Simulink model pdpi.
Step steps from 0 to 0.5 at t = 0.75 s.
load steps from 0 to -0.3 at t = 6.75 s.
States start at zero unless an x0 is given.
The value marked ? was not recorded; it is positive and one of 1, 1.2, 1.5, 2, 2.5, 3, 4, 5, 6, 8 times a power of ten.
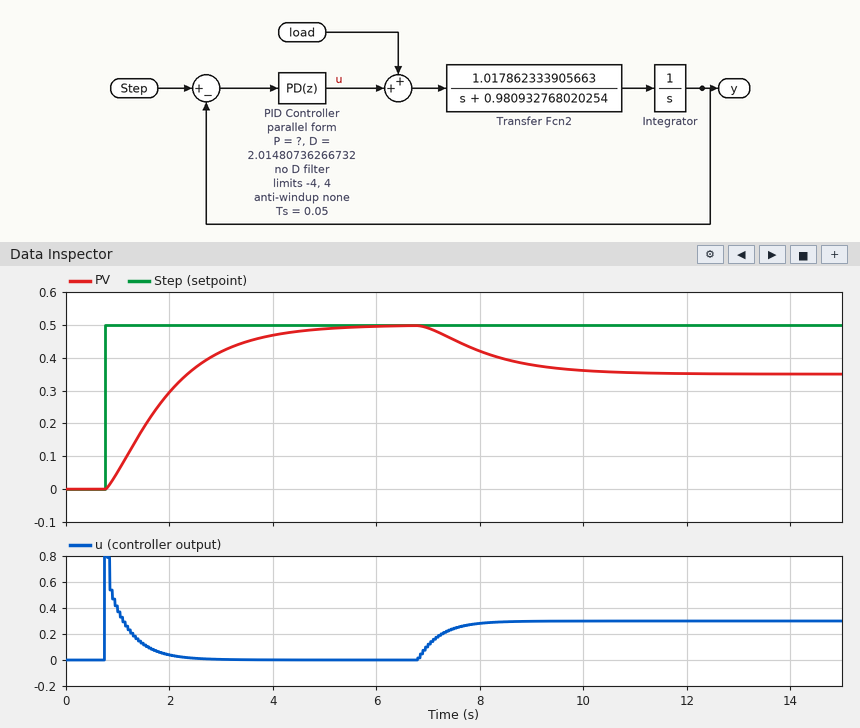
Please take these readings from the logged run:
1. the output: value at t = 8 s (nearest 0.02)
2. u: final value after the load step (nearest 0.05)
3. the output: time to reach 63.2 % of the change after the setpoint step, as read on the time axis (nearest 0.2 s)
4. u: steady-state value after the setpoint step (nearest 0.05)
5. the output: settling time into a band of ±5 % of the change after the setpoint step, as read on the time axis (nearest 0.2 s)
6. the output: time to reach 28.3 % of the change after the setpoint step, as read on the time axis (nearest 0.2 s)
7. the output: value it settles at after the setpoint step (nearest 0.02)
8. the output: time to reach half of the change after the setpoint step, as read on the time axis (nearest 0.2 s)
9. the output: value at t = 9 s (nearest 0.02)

0.42
0.30
2.2 s
0.00
4.2 s
1.4 s
0.50
1.8 s
0.38
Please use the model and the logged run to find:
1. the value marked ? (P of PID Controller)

2
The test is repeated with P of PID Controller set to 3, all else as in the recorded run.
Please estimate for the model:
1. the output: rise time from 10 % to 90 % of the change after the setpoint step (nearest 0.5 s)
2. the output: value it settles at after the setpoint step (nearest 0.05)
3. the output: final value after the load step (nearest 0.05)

1.5 s
0.50
0.40
